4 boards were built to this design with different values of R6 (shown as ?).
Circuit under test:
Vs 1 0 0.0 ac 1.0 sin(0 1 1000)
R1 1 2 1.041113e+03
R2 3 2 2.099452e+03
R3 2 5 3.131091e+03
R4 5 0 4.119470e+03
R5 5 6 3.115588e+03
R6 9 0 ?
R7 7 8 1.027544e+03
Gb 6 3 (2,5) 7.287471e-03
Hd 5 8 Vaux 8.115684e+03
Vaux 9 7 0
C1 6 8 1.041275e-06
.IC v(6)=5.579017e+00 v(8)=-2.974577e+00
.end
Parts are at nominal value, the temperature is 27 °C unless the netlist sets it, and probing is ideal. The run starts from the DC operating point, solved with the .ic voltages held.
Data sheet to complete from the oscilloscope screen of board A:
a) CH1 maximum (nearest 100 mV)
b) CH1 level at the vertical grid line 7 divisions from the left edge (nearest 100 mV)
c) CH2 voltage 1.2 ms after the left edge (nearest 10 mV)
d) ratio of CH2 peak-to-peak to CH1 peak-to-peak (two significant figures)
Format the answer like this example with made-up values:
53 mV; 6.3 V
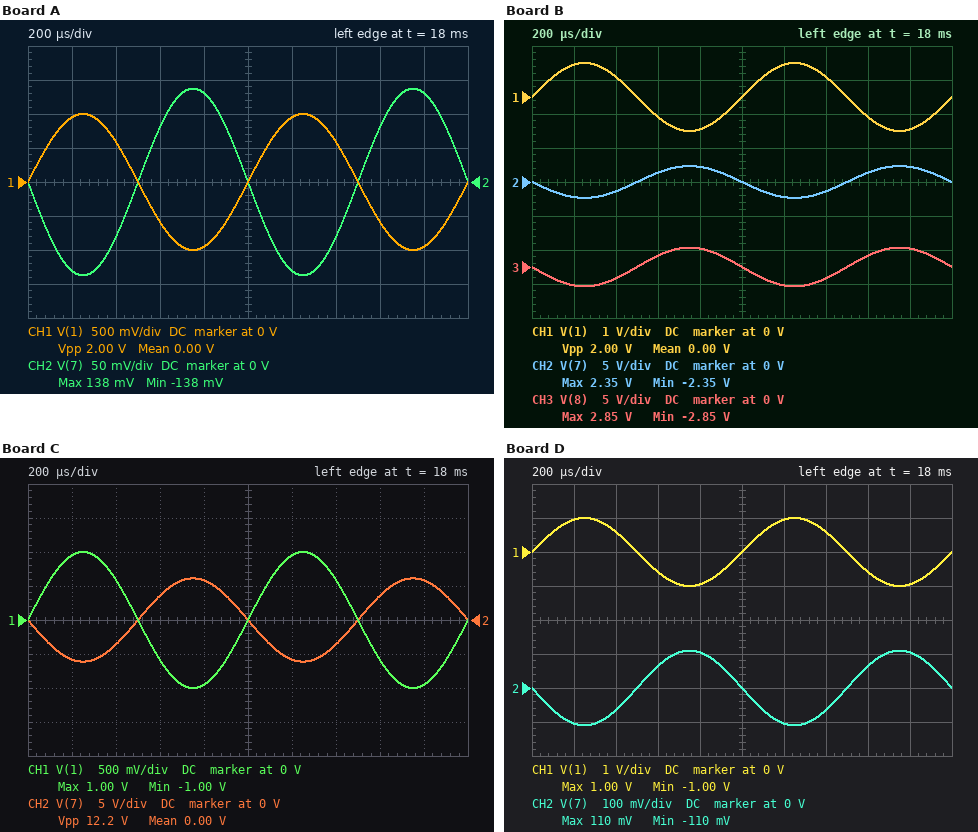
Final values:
1.0 V; 600 mV; -130 mV; 0.14
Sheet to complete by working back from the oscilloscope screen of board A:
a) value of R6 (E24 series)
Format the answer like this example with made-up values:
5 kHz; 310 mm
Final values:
910 Ω
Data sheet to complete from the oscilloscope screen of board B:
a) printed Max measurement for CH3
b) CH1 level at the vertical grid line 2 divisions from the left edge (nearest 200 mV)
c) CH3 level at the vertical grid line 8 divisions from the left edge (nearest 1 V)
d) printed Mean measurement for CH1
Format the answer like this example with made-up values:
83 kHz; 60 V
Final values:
2.85 V; 600 mV; 2 V; 0.00 V
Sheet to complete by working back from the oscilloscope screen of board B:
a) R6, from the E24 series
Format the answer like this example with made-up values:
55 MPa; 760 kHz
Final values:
4.7 kΩ
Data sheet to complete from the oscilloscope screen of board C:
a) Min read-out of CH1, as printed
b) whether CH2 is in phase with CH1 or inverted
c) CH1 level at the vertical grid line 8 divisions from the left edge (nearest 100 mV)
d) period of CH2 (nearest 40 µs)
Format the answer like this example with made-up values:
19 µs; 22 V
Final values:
-1.00 V; inverted; -600 mV; 1.00 ms
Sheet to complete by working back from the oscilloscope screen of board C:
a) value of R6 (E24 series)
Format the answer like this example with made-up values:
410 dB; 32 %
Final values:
5.6 kΩ
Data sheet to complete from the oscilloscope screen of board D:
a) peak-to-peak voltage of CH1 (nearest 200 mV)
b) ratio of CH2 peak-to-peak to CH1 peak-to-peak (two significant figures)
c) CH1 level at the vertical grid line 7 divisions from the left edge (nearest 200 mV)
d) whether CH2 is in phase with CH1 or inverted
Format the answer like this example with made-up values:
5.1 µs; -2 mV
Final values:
2.0 V; 0.11; 600 mV; inverted
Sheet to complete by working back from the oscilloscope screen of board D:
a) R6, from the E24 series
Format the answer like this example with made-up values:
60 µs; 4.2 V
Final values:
750 Ω
